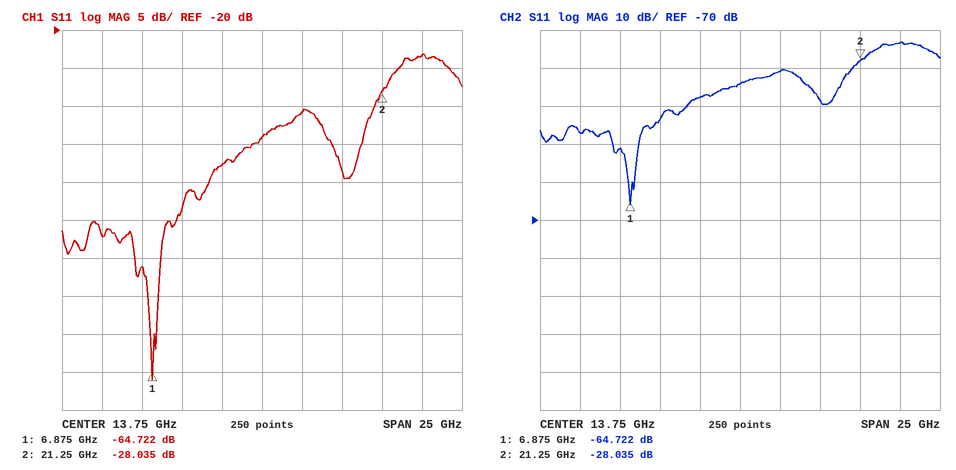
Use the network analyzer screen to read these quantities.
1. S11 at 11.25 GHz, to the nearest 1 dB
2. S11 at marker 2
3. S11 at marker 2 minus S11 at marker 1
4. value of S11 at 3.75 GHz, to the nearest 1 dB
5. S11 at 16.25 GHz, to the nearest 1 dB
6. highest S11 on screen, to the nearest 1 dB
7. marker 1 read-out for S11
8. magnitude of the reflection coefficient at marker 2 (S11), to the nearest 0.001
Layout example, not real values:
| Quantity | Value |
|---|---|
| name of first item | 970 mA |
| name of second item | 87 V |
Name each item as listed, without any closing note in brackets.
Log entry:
| Quantity | Value |
|---|---|
| S11 at 11.25 GHz, to the nearest 1 dB | -38 dB |
| S11 at marker 2 | -28.035 dB |
| S11 at marker 2 minus S11 at marker 1 | 36.687 dB |
| value of S11 at 3.75 GHz, to the nearest 1 dB | -47 dB |
| S11 at 16.25 GHz, to the nearest 1 dB | -31 dB |
| highest S11 on screen, to the nearest 1 dB | -23 dB |
| marker 1 read-out for S11 | -64.722 dB |
| magnitude of the reflection coefficient at marker 2 (S11), to the nearest 0.001 | 0.040 |
